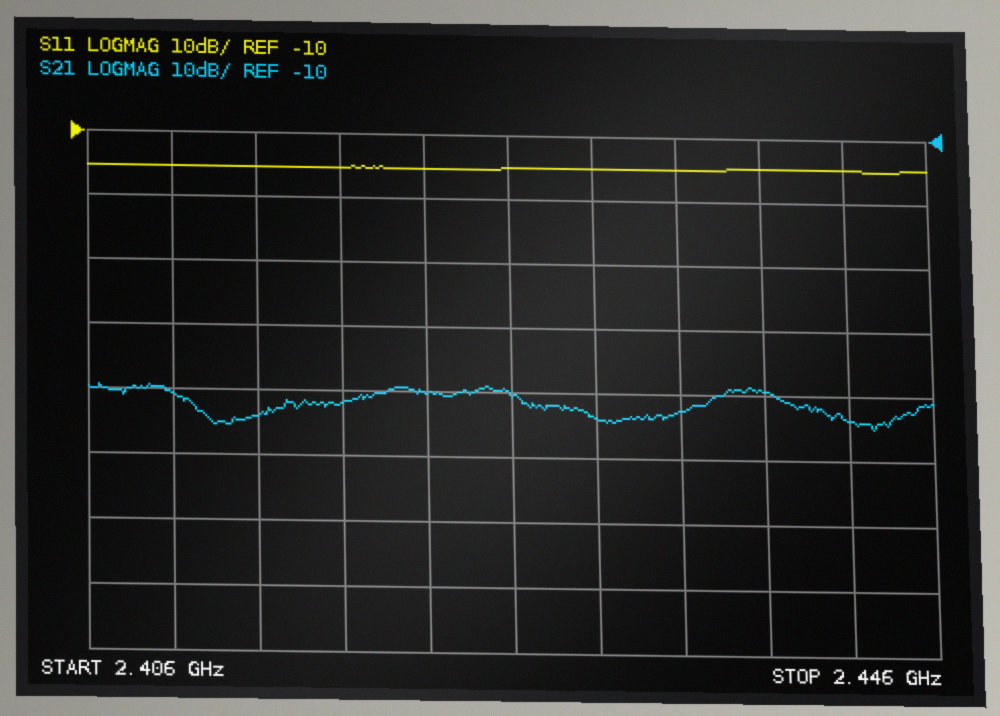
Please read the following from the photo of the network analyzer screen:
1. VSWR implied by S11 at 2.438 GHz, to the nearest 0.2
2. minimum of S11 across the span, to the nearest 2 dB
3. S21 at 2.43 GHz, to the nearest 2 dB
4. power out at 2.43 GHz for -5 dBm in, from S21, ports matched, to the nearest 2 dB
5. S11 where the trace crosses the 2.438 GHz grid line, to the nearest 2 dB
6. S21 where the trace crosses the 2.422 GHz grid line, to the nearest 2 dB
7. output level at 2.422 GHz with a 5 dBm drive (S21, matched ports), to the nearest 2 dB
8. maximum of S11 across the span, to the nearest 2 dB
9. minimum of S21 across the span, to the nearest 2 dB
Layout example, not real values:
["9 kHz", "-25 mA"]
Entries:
["1.4", "-16 dB", "-54 dB", "-58 dBm", "-14 dB", "-50 dB", "-46 dBm", "-14 dB", "-56 dB"]
